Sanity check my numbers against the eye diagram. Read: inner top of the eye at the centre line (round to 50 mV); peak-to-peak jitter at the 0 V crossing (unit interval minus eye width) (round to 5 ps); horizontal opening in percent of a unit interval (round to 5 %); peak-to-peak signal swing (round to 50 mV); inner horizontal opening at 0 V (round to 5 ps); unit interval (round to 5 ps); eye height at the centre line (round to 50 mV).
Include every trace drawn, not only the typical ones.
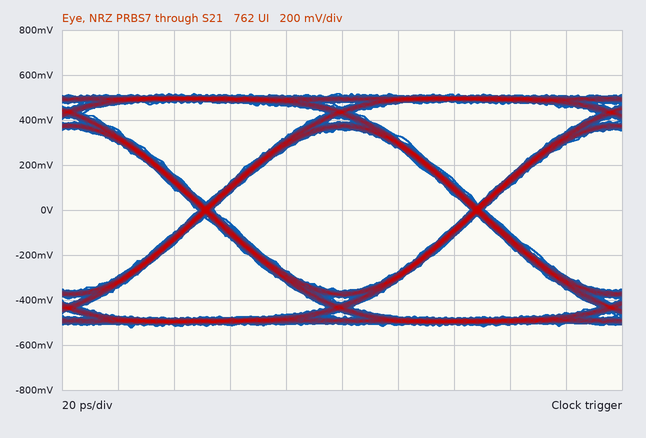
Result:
350 mV
5 ps
95 %
1.05 V
90 ps
95 ps
700 mV
